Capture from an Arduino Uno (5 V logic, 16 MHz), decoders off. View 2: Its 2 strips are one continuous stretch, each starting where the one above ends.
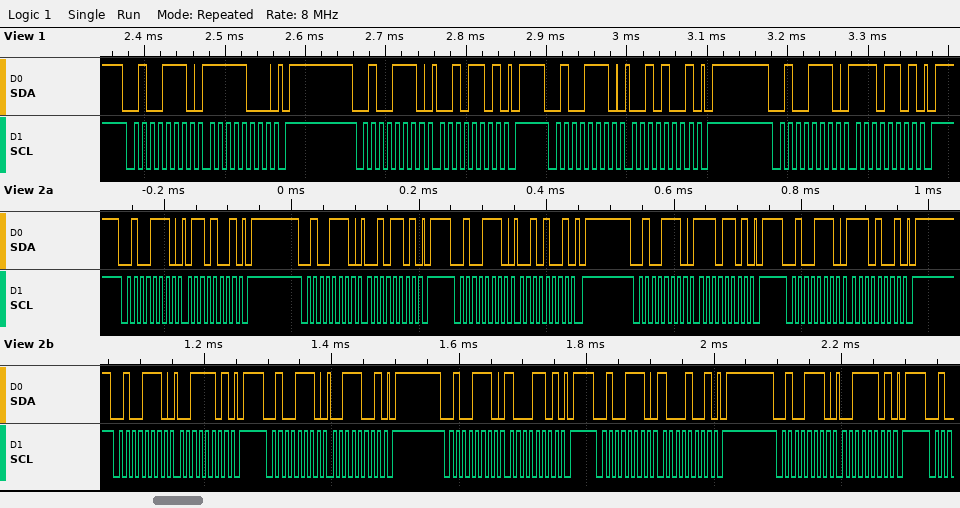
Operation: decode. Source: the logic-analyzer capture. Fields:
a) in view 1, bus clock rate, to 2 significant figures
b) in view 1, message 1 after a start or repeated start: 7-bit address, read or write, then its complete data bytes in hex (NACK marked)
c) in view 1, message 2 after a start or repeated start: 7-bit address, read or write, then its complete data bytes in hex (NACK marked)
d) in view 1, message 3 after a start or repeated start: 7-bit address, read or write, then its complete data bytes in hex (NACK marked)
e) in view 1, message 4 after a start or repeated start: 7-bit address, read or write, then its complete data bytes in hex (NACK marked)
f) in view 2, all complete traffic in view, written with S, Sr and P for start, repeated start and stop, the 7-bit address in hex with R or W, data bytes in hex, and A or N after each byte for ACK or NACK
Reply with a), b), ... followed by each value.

a) 100 kHz
b) 0x27 write: F8
c) 0x27 write: 2D
d) 0x27 write: 29
e) 0x27 write: ED
f) S 27W A 69 A P S 27W A 2D A P S 27W A 29 A P S 27W A ED A P S 27W A E9 A P S 27W A 3D A P S 27W A 39 A P S 27W A 8D A P S 27W A 89 A P S 27W A 3D A P
